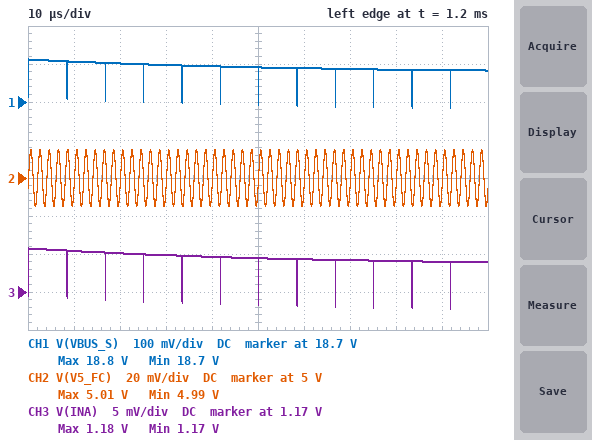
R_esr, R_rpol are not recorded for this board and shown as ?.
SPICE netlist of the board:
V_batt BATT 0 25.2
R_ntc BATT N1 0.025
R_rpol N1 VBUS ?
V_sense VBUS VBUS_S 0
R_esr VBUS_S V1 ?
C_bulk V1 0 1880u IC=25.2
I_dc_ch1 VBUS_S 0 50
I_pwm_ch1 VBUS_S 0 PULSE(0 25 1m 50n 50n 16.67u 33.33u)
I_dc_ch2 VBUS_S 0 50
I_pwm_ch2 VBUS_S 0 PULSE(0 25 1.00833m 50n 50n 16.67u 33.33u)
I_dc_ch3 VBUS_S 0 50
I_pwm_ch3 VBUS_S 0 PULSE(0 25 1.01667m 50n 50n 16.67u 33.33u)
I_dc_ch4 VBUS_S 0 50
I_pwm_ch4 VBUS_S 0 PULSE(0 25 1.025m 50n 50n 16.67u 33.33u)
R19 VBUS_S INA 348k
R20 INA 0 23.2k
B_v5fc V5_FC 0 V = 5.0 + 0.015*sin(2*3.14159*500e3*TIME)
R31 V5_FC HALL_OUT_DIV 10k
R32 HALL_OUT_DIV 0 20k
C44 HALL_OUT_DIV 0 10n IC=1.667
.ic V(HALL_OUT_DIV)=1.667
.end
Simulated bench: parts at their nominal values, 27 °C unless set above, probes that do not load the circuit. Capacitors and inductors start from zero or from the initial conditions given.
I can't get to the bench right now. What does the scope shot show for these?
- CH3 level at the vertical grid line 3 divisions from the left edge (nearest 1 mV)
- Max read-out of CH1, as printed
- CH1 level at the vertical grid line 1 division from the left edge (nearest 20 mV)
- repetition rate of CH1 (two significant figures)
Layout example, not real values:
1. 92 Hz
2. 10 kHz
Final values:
1. 1.175 V
2. 18.8 V
3. 18.80 V
4. 120 kHz
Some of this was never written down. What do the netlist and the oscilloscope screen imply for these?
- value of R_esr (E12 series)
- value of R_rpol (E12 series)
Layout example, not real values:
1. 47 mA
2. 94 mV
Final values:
1. 4.7 mΩ
2. 680 µΩ
